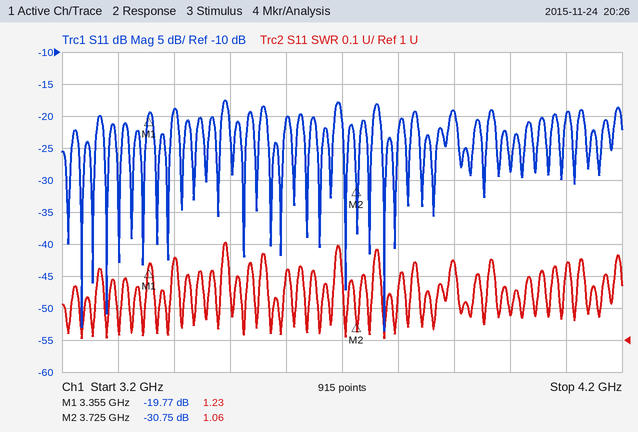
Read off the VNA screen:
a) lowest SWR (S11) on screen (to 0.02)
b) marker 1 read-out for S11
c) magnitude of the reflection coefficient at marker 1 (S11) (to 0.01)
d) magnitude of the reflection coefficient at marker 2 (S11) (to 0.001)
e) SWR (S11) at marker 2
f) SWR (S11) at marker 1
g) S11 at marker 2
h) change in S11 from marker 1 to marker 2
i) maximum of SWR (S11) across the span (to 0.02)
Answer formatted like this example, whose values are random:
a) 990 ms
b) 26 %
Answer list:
a) 1.00
b) -19.77 dB
c) 0.10
d) 0.029
e) 1.06
f) 1.23
g) -30.75 dB
h) -10.98 dB
i) 1.30
